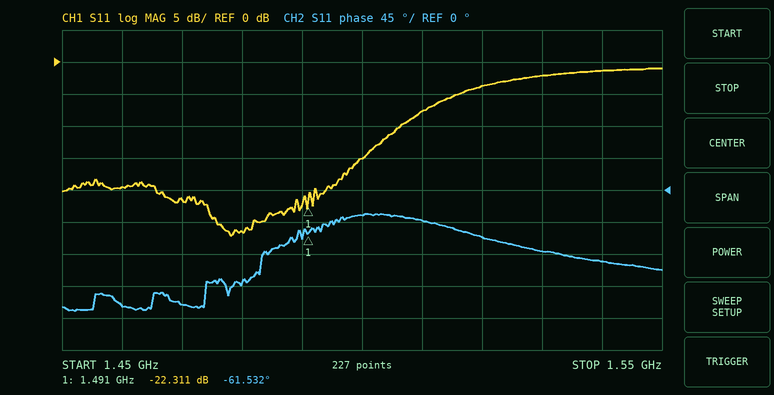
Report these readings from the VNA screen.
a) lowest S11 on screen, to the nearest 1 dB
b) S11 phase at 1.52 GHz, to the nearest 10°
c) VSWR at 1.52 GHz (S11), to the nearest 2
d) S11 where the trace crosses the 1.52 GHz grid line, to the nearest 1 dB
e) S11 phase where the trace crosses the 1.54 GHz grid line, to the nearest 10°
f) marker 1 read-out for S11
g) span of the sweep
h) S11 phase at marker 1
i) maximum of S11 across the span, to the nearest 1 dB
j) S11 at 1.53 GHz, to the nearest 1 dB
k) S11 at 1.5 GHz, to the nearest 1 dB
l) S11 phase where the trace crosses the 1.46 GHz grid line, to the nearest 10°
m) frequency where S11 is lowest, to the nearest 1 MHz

-27 dB
-70°
4
-4 dB
-100°
-22.311 dB
100 MHz
-61.532°
-1 dB
-2 dB
-15 dB
-160°
1.478 GHz
